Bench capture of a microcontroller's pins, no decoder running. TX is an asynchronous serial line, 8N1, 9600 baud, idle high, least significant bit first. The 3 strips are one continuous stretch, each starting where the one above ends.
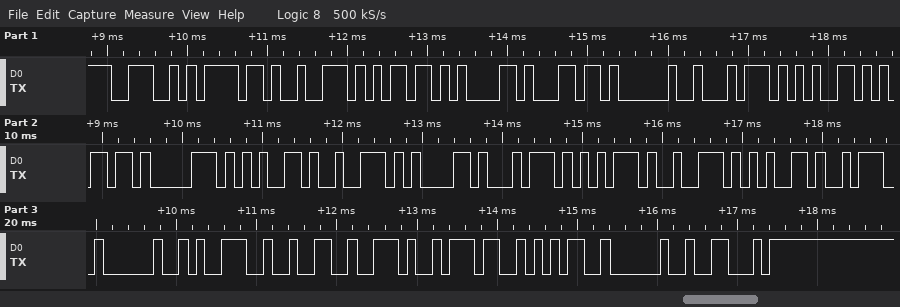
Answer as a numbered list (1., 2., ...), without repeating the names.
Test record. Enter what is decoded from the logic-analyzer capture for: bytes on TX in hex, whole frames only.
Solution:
1. 4E 6F 72 6D 61 6C 20 74 65 6D 70 65 72 61 74 75 72 65 3A 20 39 32 2E 37 35 20 46
